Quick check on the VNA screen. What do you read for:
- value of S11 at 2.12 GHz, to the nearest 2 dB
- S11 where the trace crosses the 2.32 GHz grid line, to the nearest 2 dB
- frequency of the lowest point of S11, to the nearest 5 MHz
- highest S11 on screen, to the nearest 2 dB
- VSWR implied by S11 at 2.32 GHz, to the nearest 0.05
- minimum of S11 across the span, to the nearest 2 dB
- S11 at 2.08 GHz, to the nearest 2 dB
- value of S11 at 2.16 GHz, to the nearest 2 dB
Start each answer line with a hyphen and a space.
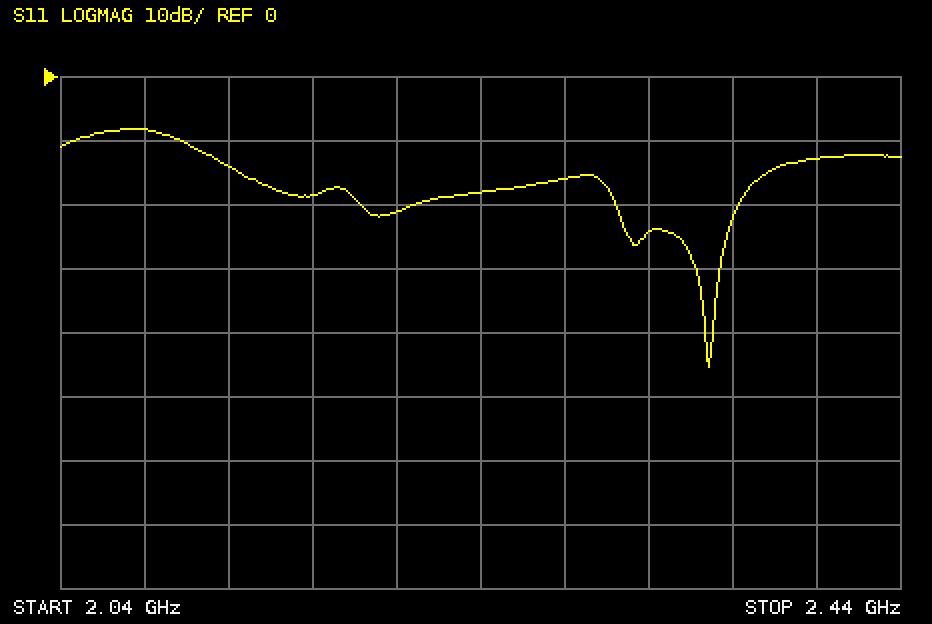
- -14 dB
- -24 dB
- 2.350 GHz
- -8 dB
- 1.15
- -46 dB
- -8 dB
- -18 dB
